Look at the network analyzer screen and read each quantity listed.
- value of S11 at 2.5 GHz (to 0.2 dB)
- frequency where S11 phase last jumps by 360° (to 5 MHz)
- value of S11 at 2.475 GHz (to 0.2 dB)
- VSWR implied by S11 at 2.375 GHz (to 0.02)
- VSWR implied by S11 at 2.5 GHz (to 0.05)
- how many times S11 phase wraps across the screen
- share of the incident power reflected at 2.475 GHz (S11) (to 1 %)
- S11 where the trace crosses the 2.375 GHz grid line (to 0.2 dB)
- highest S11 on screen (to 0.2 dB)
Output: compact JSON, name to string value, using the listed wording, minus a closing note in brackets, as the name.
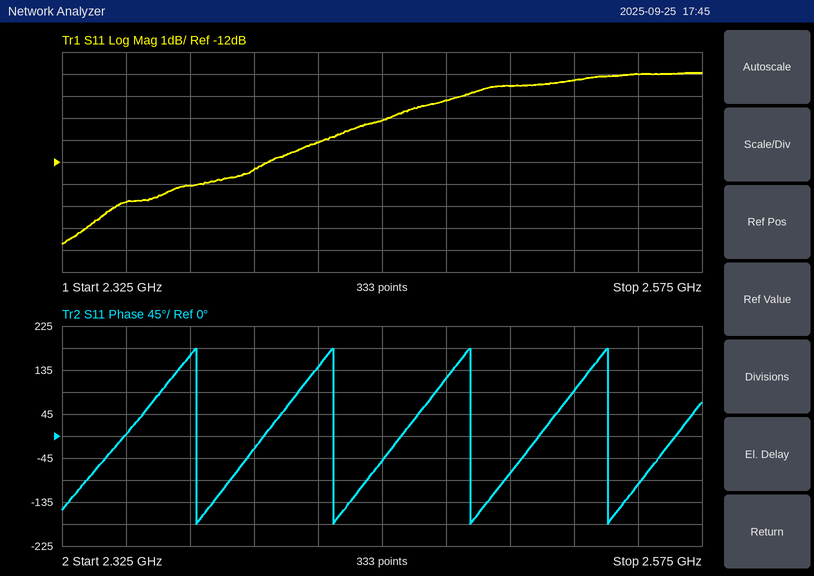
{"value of S11 at 2.5 GHz": "-8.6 dB", "frequency where S11 phase last jumps by 360°": "2.540 GHz", "value of S11 at 2.475 GHz": "-9.2 dB", "VSWR implied by S11 at 2.375 GHz": "1.58", "VSWR implied by S11 at 2.5 GHz": "2.20", "how many times S11 phase wraps across the screen": "4", "share of the incident power reflected at 2.475 GHz (S11)": "12 %", "S11 where the trace crosses the 2.375 GHz grid line": "-13.0 dB", "highest S11 on screen": "-8.0 dB"}
